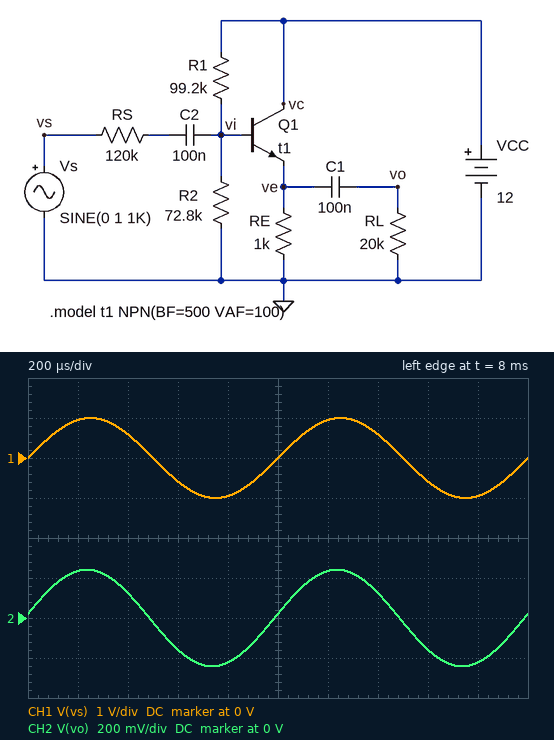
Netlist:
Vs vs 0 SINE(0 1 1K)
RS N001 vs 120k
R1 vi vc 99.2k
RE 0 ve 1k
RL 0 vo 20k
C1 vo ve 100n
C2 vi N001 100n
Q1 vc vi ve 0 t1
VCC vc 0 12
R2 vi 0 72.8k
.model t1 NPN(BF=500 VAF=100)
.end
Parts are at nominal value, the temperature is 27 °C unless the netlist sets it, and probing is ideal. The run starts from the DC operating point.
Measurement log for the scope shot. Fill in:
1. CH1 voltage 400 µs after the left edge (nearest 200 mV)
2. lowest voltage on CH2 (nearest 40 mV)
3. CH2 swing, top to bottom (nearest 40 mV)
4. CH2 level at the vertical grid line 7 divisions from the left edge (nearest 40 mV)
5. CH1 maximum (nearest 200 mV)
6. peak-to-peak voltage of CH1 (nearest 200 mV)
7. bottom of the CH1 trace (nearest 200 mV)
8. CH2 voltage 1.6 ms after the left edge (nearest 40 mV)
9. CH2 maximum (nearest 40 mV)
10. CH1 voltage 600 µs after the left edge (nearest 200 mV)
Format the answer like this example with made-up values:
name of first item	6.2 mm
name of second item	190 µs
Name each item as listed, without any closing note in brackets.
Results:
CH1 voltage 400 µs after the left edge	600 mV
lowest voltage on CH2	-240 mV
CH2 swing, top to bottom	480 mV
CH2 level at the vertical grid line 7 divisions from the left edge	120 mV
CH1 maximum	1.0 V
peak-to-peak voltage of CH1	2.0 V
bottom of the CH1 trace	-1.0 V
CH2 voltage 1.6 ms after the left edge	-160 mV
CH2 maximum	240 mV
CH1 voltage 600 µs after the left edge	-600 mV
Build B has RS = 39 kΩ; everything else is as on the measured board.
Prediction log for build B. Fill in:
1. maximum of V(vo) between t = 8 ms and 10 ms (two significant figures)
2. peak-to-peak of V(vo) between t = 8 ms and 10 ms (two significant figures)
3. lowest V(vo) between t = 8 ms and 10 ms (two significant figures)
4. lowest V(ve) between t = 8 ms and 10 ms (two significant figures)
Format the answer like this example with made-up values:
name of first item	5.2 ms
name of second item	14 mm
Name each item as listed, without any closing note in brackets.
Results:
maximum of V(vo) between t = 8 ms and 10 ms	490 mV
peak-to-peak of V(vo) between t = 8 ms and 10 ms	990 mV
lowest V(vo) between t = 8 ms and 10 ms	-490 mV
lowest V(ve) between t = 8 ms and 10 ms	3.5 V
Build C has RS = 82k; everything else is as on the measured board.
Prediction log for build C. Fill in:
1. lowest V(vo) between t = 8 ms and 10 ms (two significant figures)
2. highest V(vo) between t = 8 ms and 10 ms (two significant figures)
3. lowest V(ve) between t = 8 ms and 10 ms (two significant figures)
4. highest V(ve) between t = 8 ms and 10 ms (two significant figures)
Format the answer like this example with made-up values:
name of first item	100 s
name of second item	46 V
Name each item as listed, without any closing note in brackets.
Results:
lowest V(vo) between t = 8 ms and 10 ms	-320 mV
highest V(vo) between t = 8 ms and 10 ms	320 mV
lowest V(ve) between t = 8 ms and 10 ms	3.6 V
highest V(ve) between t = 8 ms and 10 ms	4.3 V
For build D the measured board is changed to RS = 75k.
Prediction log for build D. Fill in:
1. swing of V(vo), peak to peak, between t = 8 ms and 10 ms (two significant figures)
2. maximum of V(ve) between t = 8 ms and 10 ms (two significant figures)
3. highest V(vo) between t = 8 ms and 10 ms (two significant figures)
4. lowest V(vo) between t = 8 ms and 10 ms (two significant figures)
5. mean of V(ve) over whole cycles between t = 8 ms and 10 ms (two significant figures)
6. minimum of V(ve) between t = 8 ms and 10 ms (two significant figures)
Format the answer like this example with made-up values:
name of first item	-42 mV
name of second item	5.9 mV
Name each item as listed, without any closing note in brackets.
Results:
swing of V(vo), peak to peak, between t = 8 ms and 10 ms	670 mV
maximum of V(ve) between t = 8 ms and 10 ms	4.3 V
highest V(vo) between t = 8 ms and 10 ms	340 mV
lowest V(vo) between t = 8 ms and 10 ms	-340 mV
mean of V(ve) over whole cycles between t = 8 ms and 10 ms	4.0 V
minimum of V(ve) between t = 8 ms and 10 ms	3.6 V
